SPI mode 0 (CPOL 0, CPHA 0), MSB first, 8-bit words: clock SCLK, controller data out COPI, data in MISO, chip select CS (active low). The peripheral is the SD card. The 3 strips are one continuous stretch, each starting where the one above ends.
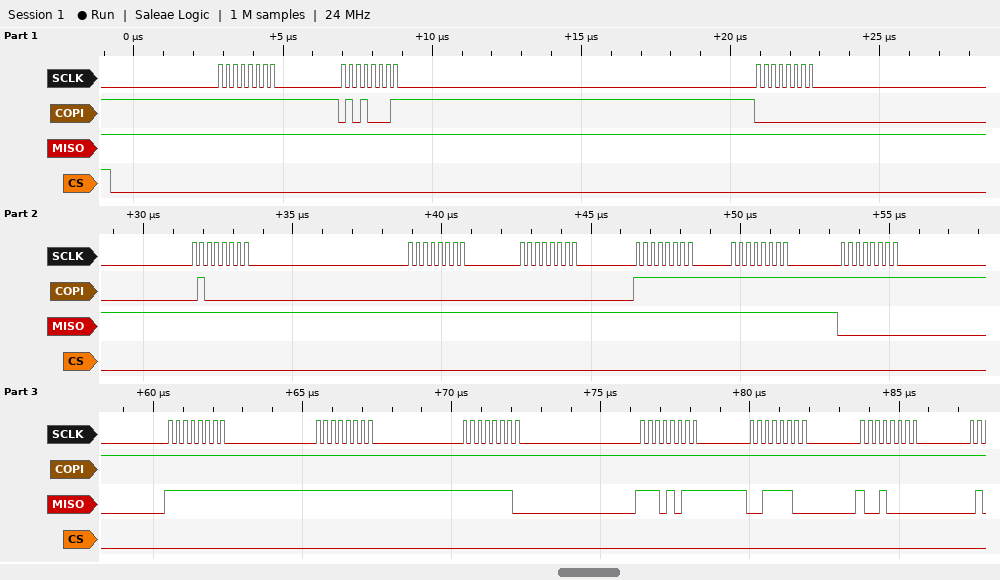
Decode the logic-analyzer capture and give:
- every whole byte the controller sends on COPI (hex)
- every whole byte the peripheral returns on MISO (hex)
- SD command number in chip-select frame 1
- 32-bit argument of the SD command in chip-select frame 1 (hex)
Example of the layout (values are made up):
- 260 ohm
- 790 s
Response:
- FF 51 00 40 00 00 FF FF FF FF FF FF FF FF FF
- FF FF FF FF FF FF FF FF 00 FF FF FE EB 3C 90
- CMD17
- 0x00400000
